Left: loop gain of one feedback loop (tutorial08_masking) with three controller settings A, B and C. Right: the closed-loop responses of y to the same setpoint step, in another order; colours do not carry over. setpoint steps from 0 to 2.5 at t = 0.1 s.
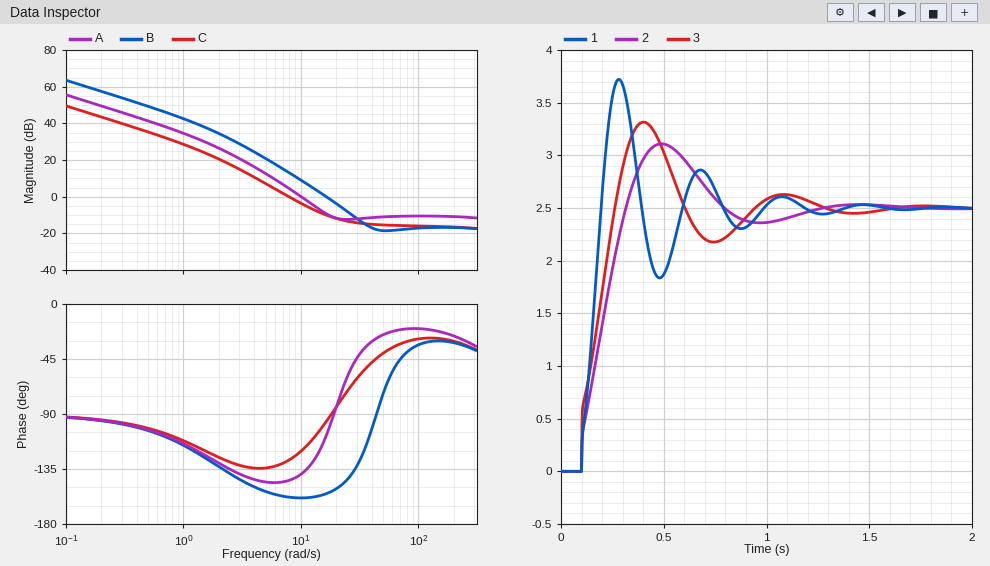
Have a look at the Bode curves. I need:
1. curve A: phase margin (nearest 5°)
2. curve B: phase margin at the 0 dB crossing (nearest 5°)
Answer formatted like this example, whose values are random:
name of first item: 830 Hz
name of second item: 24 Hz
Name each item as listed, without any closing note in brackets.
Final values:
curve A: phase margin: 40°
curve B: phase margin at the 0 dB crossing: 25°
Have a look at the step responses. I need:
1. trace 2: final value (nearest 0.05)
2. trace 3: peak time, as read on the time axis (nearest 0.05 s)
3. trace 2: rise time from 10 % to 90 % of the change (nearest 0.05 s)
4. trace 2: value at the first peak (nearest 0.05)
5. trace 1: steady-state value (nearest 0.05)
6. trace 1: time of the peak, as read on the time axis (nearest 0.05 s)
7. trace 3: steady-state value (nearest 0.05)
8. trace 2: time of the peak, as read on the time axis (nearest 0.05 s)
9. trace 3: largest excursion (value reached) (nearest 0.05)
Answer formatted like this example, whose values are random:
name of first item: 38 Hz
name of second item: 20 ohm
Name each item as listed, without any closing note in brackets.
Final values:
trace 2: final value: 2.50
trace 3: peak time, as read on the time axis: 0.40 s
trace 2: rise time from 10 % to 90 % of the change: 0.20 s
trace 2: value at the first peak: 3.10
trace 1: steady-state value: 2.50
trace 1: time of the peak, as read on the time axis: 0.30 s
trace 3: steady-state value: 2.50
trace 2: time of the peak, as read on the time axis: 0.50 s
trace 3: largest excursion (value reached): 3.30
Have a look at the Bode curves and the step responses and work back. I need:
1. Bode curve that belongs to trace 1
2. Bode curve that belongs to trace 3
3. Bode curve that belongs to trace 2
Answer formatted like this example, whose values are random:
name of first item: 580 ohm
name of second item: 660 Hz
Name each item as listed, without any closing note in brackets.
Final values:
Bode curve that belongs to trace 1: B
Bode curve that belongs to trace 3: A
Bode curve that belongs to trace 2: C
